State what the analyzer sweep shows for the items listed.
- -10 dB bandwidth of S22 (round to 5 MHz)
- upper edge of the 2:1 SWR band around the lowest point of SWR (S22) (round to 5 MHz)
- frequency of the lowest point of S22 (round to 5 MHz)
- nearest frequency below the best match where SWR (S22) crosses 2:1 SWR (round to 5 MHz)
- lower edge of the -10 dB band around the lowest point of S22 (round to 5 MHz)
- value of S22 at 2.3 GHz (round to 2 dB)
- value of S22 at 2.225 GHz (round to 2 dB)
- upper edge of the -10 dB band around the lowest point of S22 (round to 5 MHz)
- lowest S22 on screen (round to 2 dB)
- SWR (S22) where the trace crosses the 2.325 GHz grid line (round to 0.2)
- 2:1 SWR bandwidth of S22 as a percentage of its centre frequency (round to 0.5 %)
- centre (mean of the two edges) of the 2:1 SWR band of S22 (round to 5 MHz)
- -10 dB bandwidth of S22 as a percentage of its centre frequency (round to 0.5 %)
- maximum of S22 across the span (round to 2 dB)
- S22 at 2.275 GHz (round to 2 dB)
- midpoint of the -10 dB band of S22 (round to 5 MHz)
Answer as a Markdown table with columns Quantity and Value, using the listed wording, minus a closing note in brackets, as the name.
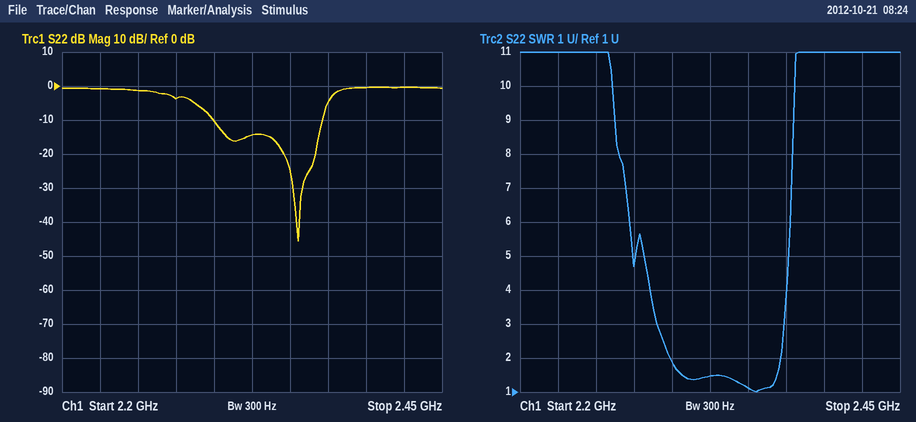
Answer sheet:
| Quantity | Value |
|---|---|
| -10 dB bandwidth of S22 | 70 MHz |
| upper edge of the 2:1 SWR band around the lowest point of SWR (S22) | 2.370 GHz |
| frequency of the lowest point of S22 | 2.355 GHz |
| nearest frequency below the best match where SWR (S22) crosses 2:1 SWR | 2.300 GHz |
| lower edge of the -10 dB band around the lowest point of S22 | 2.300 GHz |
| value of S22 at 2.3 GHz | -10 dB |
| value of S22 at 2.225 GHz | 0 dB |
| upper edge of the -10 dB band around the lowest point of S22 | 2.370 GHz |
| lowest S22 on screen | -46 dB |
| SWR (S22) where the trace crosses the 2.325 GHz grid line | 1.4 |
| 2:1 SWR bandwidth of S22 as a percentage of its centre frequency | 3.0 % |
| centre (mean of the two edges) of the 2:1 SWR band of S22 | 2.335 GHz |
| -10 dB bandwidth of S22 as a percentage of its centre frequency | 3.0 % |
| maximum of S22 across the span | 0 dB |
| S22 at 2.275 GHz | -4 dB |
| midpoint of the -10 dB band of S22 | 2.335 GHz |
